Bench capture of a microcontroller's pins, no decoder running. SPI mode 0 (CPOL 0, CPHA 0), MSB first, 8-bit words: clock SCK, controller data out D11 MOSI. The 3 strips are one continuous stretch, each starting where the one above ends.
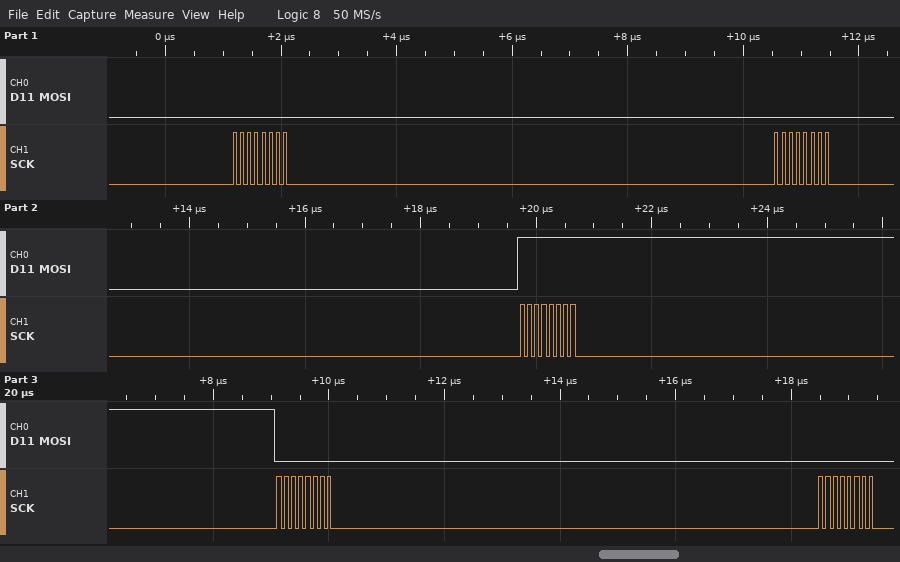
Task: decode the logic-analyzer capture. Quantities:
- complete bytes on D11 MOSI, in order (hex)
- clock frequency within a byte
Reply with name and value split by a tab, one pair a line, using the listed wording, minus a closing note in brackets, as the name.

complete bytes on D11 MOSI, in order	00 00 FF 00 00
clock frequency within a byte	8 MHz
